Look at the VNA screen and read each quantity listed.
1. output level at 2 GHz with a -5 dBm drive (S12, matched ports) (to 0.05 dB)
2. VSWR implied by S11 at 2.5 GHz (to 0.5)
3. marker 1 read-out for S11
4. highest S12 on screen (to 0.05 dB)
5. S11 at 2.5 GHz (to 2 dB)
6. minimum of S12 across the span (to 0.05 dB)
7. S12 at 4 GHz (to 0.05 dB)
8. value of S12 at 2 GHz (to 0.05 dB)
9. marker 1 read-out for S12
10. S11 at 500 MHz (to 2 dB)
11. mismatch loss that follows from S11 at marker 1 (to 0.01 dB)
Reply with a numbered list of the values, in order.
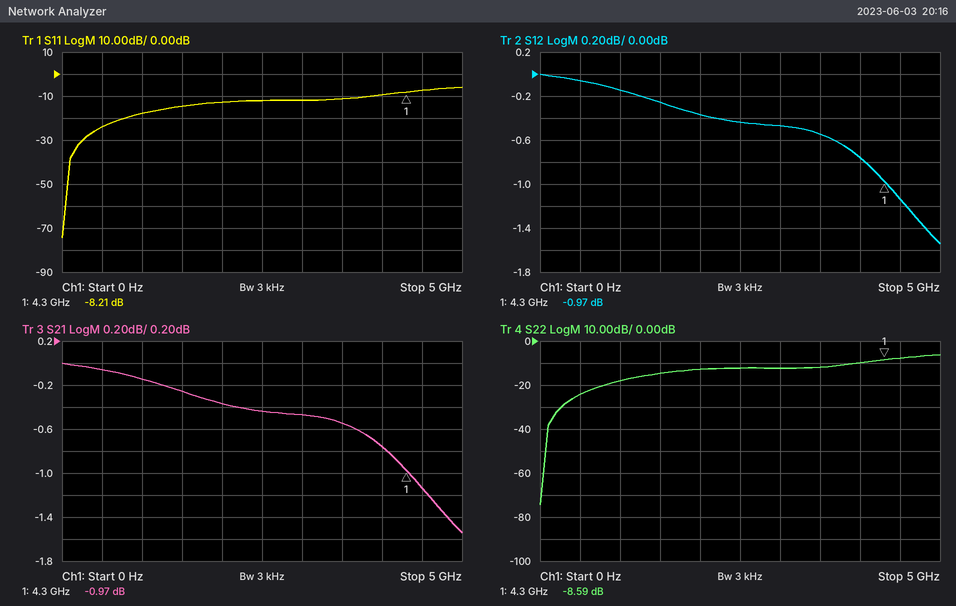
1. -5.35 dBm
2. 1.5
3. -8.21 dB
4. 0.00 dB
5. -12 dB
6. -1.55 dB
7. -0.75 dB
8. -0.35 dB
9. -0.97 dB
10. -24 dB
11. 0.71 dB
